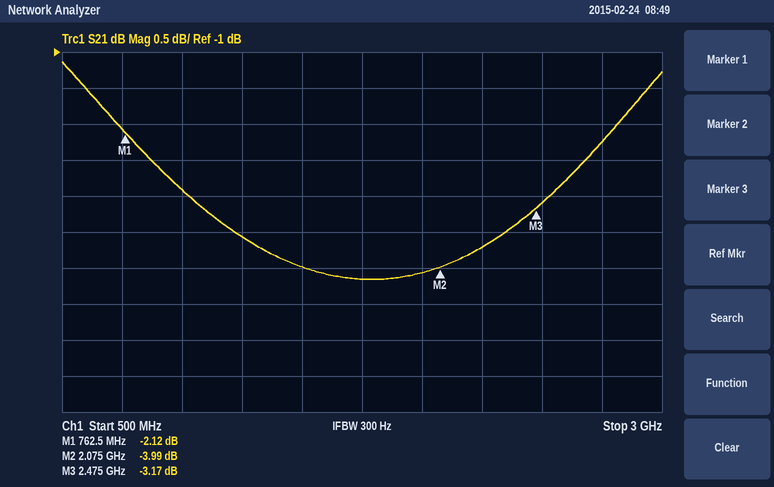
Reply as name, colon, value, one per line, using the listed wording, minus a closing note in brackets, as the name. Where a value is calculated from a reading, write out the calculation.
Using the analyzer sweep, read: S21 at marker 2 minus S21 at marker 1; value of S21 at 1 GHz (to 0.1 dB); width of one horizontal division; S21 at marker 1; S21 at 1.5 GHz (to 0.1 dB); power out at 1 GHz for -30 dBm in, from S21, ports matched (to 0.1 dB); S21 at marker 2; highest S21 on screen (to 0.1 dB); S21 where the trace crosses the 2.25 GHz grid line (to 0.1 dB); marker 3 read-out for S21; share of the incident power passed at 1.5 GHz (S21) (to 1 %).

S21 at marker 2 minus S21 at marker 1: -3.99 − (-2.12) = -1.87 dB
value of S21 at 1 GHz: -2.9 dB
width of one horizontal division: 250 MHz
S21 at marker 1: -2.12 dB
S21 at 1.5 GHz: -4.0 dB
power out at 1 GHz for -30 dBm in, from S21, ports matched: -30 dBm + (-2.9 dB) = -32.9 dBm
S21 at marker 2: -3.99 dB
highest S21 on screen: -1.1 dB
S21 where the trace crosses the 2.25 GHz grid line: -3.7 dB
marker 3 read-out for S21: -3.17 dB
share of the incident power passed at 1.5 GHz (S21): 10^(-4/10) ≈ 40 %
